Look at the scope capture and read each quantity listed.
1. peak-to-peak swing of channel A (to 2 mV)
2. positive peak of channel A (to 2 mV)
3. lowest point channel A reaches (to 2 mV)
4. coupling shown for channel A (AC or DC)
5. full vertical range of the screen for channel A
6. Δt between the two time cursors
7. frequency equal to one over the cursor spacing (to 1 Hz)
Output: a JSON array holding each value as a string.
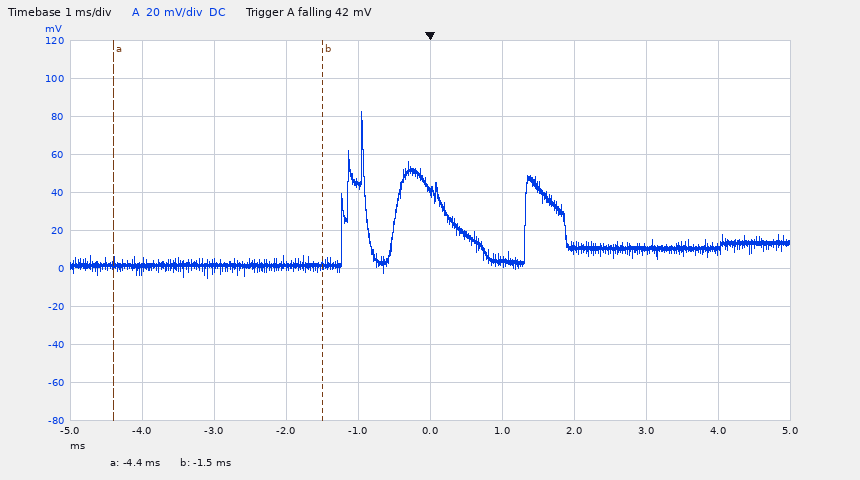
["88 mV", "82 mV", "-6 mV", "DC", "200 mV", "2.9 ms", "345 Hz"]
